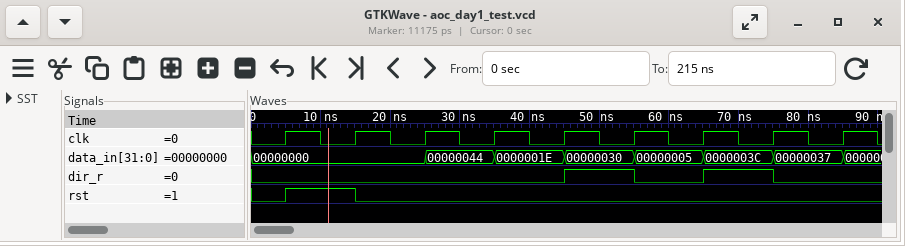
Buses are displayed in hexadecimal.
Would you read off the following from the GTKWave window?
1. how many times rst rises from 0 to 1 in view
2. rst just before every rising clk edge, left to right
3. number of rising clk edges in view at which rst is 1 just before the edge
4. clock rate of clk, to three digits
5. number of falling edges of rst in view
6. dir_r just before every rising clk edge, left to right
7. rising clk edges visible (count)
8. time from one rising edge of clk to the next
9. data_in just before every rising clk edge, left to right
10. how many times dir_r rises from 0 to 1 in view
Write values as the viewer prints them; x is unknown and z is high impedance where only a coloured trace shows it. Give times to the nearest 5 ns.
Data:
1
0 1 0 0 0 0 0 0 0
1
100 MHz
1
0 0 0 0 0 1 0 1 0
9
10 ns
00000000, 00000000, 00000000, 00000044, 0000001E, 00000030, 00000005, 0000003C, 00000037
2
